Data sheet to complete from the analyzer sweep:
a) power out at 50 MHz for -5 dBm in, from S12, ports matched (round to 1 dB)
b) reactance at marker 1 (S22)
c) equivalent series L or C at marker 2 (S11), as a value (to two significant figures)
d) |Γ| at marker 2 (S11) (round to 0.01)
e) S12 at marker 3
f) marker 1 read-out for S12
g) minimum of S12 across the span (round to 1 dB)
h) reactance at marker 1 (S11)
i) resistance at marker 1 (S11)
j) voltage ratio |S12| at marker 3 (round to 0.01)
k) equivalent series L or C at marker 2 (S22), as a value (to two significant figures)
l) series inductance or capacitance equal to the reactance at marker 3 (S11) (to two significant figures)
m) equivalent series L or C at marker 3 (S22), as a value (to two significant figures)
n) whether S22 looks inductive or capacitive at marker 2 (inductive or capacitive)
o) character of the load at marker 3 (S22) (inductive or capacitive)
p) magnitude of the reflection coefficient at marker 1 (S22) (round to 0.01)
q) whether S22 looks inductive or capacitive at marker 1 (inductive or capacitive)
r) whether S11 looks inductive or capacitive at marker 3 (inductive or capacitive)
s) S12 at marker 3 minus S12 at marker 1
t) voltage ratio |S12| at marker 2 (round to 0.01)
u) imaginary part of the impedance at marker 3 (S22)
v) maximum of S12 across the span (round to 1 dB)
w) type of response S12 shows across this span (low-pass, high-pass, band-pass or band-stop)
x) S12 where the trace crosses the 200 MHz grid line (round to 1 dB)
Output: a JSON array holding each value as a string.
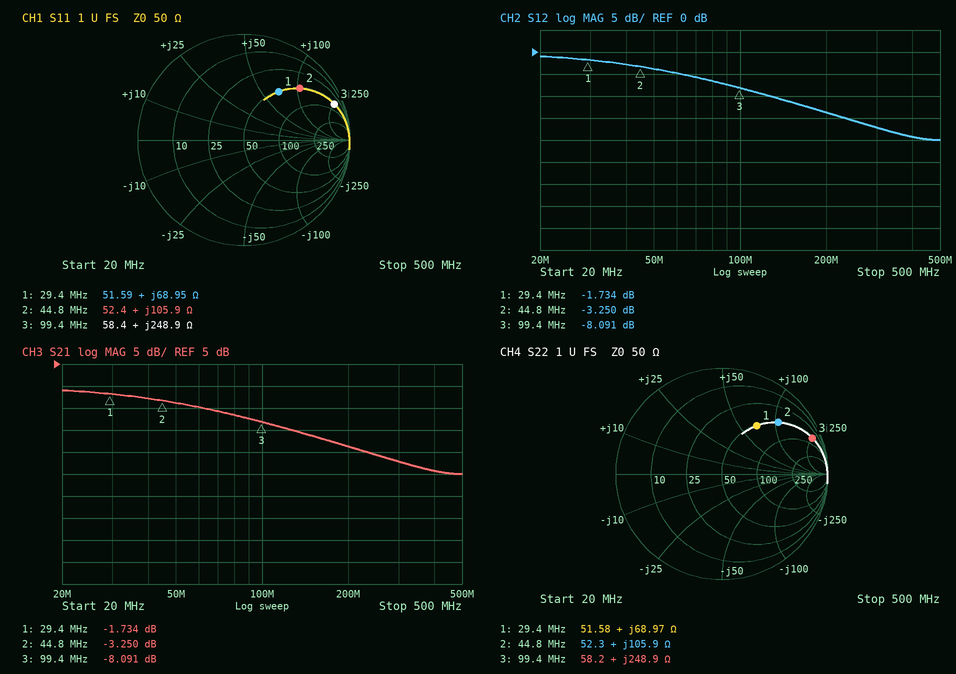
["-9 dBm", "+68.97 Ω", "380 nH", "0.72", "-8.091 dB", "-1.734 dB", "-20 dB", "+68.95 Ω", "51.59 Ω", "0.39", "380 nH", "400 nH", "400 nH", "inductive", "inductive", "0.56", "inductive", "inductive", "-6.357 dB", "0.69", "+248.9 Ω", "-1 dB", "low-pass", "-14 dB"]
